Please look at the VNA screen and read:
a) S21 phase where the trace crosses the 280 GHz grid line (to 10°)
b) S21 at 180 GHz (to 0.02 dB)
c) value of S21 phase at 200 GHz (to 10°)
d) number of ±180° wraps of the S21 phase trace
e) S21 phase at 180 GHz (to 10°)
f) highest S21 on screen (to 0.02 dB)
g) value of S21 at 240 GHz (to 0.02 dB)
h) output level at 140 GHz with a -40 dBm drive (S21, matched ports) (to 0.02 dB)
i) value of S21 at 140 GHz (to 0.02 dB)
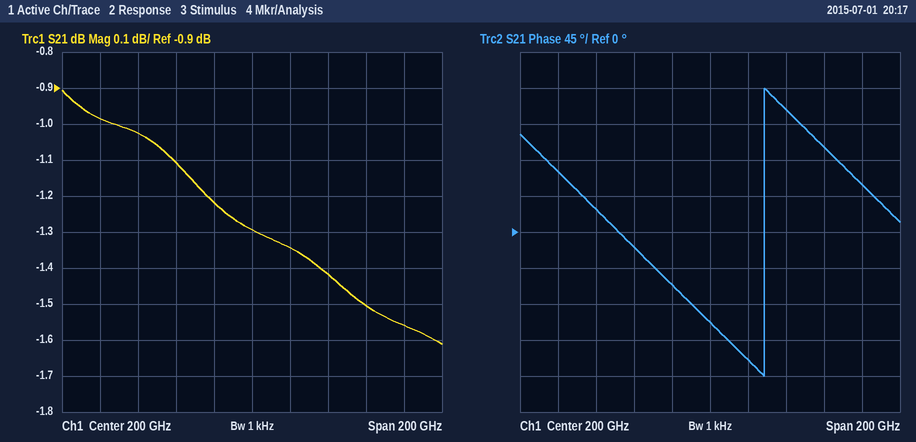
60°
-1.22 dB
-110°
1
-70°
-0.90 dB
-1.42 dB
-41.02 dBm
-1.02 dB
